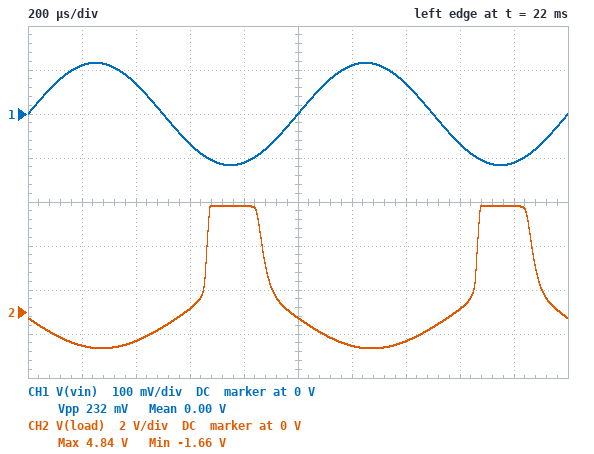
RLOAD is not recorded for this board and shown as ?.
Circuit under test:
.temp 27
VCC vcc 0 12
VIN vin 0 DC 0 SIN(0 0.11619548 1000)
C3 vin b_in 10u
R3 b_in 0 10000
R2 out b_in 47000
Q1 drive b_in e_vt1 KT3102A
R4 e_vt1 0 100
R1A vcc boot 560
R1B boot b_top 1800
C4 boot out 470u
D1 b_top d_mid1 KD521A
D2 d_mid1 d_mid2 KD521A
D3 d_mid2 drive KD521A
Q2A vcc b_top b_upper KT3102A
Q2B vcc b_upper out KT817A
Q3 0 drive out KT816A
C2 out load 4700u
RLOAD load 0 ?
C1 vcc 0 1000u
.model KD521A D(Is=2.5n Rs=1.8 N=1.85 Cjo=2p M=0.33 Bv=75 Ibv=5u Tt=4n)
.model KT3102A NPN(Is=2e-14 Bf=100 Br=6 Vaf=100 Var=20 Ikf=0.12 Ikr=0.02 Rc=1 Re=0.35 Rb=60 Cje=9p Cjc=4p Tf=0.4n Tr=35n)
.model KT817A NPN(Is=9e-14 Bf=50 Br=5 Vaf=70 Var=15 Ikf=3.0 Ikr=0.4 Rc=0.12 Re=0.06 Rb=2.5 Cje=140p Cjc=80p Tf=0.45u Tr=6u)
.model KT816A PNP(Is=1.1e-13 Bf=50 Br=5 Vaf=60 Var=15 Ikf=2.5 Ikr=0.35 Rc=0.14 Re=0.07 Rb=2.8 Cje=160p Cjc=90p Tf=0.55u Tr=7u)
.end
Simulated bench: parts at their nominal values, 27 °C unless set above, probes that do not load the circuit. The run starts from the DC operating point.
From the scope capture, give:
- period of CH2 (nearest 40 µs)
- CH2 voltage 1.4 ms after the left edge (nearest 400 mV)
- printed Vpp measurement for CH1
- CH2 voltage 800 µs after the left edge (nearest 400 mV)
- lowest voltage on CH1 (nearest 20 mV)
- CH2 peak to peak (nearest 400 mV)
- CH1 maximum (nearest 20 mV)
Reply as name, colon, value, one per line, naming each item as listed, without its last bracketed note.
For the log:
period of CH2: 1.00 ms
CH2 voltage 1.4 ms after the left edge: -1.2 V
printed Vpp measurement for CH1: 232 mV
CH2 voltage 800 µs after the left edge: 4.8 V
lowest voltage on CH1: -120 mV
CH2 peak to peak: 6.4 V
CH1 maximum: 120 mV
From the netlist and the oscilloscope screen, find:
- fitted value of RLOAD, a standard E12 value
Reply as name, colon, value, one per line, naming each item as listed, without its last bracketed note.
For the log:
fitted value of RLOAD, a standard E12 value: 22 Ω
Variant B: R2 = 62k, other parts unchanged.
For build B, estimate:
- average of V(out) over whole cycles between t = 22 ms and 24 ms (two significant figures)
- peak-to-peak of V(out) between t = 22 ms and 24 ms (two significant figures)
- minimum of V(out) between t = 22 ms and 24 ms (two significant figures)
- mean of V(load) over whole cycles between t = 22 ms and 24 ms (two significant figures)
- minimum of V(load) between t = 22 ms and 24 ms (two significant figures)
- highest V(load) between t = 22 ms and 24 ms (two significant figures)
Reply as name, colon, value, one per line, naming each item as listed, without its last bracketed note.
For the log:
average of V(out) over whole cycles between t = 22 ms and 24 ms: 7.9 V
peak-to-peak of V(out) between t = 22 ms and 24 ms: 5.5 V
minimum of V(out) between t = 22 ms and 24 ms: 5.7 V
mean of V(load) over whole cycles between t = 22 ms and 24 ms: 590 mV
minimum of V(load) between t = 22 ms and 24 ms: -1.5 V
highest V(load) between t = 22 ms and 24 ms: 3.9 V
